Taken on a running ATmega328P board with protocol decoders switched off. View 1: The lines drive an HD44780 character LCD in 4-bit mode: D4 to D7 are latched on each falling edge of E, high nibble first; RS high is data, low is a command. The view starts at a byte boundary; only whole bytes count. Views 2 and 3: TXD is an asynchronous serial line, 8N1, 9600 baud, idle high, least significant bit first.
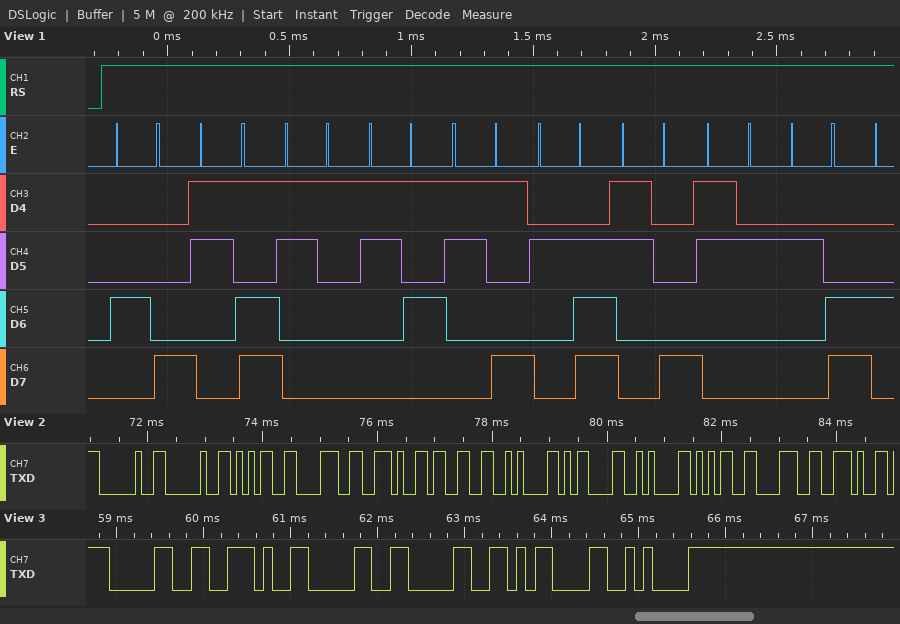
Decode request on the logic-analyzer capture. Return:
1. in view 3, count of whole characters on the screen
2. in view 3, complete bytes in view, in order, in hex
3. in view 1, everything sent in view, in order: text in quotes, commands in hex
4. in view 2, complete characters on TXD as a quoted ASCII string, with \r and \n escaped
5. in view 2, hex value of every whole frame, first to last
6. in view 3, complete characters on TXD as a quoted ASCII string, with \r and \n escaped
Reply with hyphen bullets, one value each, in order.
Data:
- 6
- 0x30 0x2E 0x30 0x30 0x0D 0x0A
- "H=159.82,"
- "  58.3\n\r\n58."
- 20 20 35 38 2E 33 0A 0D 0A 35 38 2E
- "0.00\r\n"
